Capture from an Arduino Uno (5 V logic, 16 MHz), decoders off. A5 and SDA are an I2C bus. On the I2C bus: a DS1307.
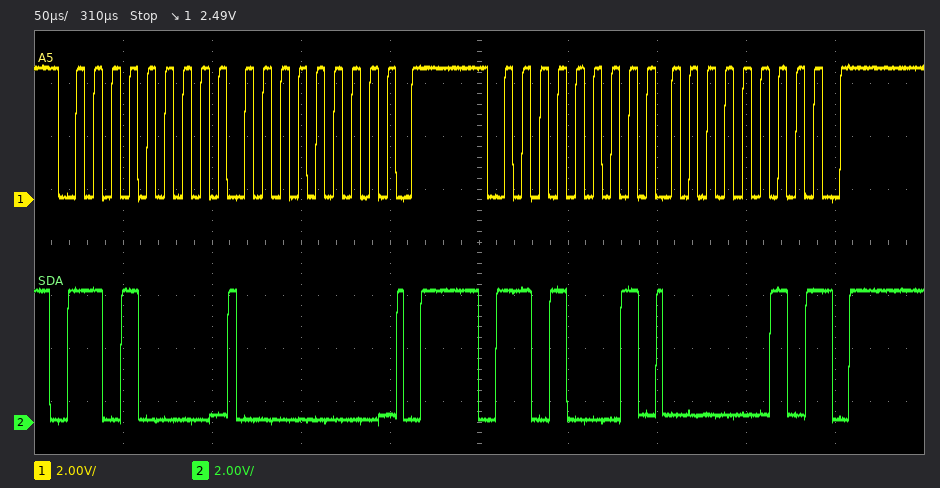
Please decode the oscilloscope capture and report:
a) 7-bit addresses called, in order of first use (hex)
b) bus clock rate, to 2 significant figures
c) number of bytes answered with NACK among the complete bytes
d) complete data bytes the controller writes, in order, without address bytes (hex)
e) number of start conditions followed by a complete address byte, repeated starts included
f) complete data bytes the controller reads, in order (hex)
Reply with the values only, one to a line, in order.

0x68
100 kHz
1
00
2
02
